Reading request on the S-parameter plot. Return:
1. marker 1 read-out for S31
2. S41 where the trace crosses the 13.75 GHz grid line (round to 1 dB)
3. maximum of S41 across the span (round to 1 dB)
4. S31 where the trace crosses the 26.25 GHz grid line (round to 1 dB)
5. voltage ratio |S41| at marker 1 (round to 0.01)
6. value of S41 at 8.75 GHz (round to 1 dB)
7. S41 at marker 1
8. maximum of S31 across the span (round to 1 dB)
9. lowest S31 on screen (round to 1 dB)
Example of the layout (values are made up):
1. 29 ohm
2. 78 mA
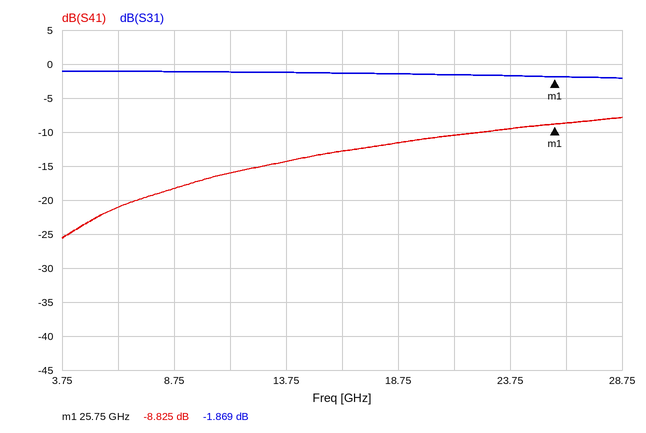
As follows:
1. -1.869 dB
2. -14 dB
3. -8 dB
4. -2 dB
5. 0.36
6. -18 dB
7. -8.825 dB
8. -1 dB
9. -2 dB
